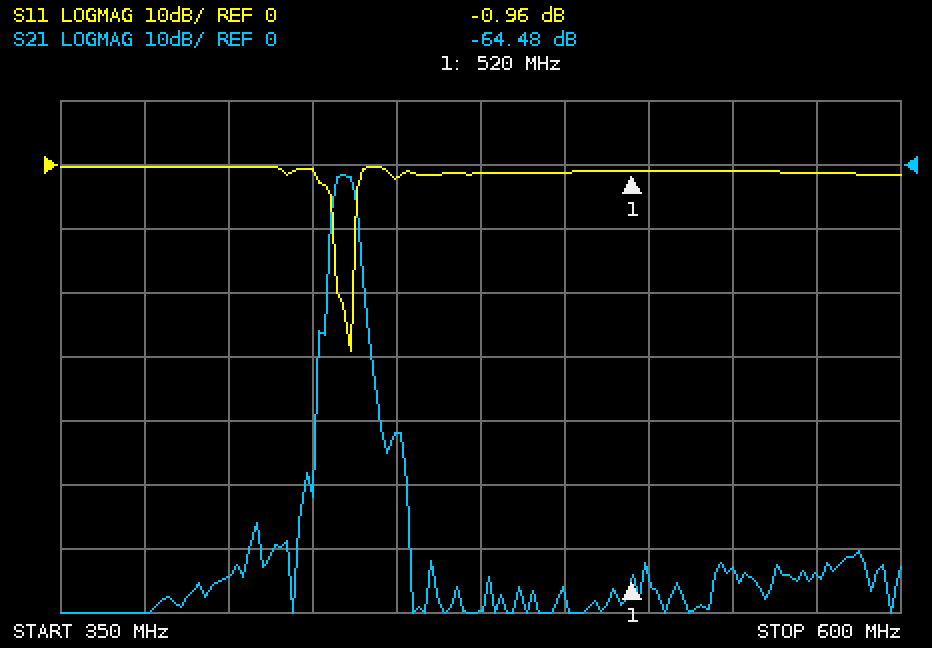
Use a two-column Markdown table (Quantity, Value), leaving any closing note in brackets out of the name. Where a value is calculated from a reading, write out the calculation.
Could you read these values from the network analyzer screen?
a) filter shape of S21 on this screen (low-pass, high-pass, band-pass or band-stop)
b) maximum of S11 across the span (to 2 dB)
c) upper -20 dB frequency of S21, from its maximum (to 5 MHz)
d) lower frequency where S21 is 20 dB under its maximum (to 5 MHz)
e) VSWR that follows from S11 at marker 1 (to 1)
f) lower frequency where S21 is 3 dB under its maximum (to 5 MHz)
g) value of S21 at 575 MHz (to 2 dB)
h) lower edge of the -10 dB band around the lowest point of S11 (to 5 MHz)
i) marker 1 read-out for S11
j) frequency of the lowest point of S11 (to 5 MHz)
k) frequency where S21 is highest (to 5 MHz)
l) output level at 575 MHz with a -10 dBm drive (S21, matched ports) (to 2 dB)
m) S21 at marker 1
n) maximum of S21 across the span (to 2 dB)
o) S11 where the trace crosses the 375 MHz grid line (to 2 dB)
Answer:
| Quantity | Value |
|---|---|
| filter shape of S21 on this screen | band-pass |
| maximum of S11 across the span | 0 dB |
| upper -20 dB frequency of S21, from its maximum | 440 MHz |
| lower frequency where S21 is 20 dB under its maximum | 430 MHz |
| VSWR that follows from S11 at marker 1 | (1 + 0.8954)/(1 − 0.8954) ≈ 18 |
| lower frequency where S21 is 3 dB under its maximum | 430 MHz |
| value of S21 at 575 MHz | -64 dB |
| lower edge of the -10 dB band around the lowest point of S11 | 430 MHz |
| marker 1 read-out for S11 | -0.96 dB |
| frequency of the lowest point of S11 | 435 MHz |
| frequency where S21 is highest | 435 MHz |
| output level at 575 MHz with a -10 dBm drive (S21, matched ports) | -10 dBm + (-64 dB) = -74 dBm |
| S21 at marker 1 | -64.48 dB |
| maximum of S21 across the span | -2 dB |
| S11 where the trace crosses the 375 MHz grid line | 0 dB |
